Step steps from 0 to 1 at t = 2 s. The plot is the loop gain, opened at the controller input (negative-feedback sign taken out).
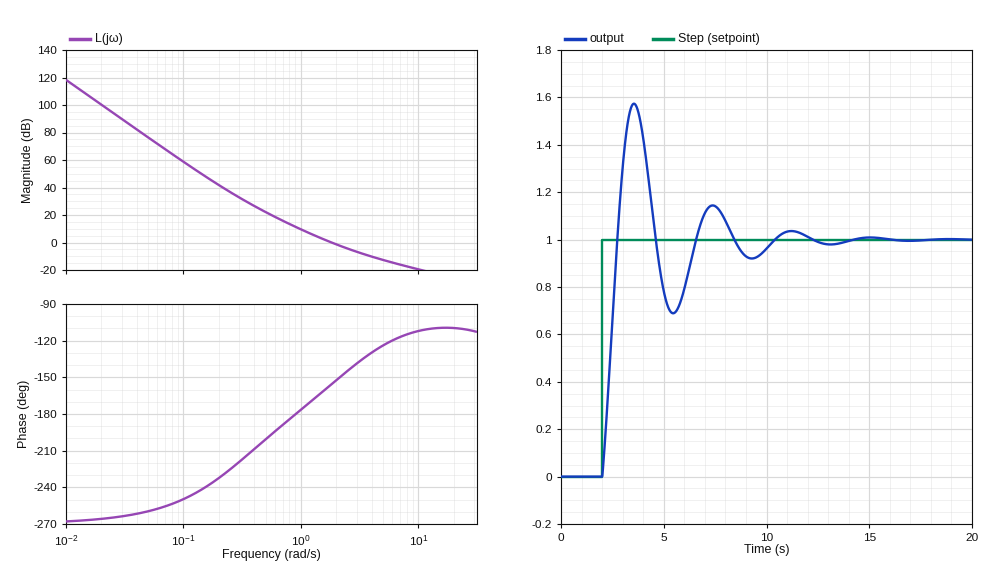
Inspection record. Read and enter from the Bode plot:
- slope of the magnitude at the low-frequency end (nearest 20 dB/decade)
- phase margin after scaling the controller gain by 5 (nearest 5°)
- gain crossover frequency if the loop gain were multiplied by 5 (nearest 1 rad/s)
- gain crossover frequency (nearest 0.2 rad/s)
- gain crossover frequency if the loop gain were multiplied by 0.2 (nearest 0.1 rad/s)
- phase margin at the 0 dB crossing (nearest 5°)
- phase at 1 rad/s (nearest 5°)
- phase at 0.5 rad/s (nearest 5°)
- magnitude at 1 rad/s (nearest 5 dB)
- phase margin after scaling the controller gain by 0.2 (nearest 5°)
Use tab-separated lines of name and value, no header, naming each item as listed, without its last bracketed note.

slope of the magnitude at the low-frequency end	-60 dB/decade
phase margin after scaling the controller gain by 5	60°
gain crossover frequency if the loop gain were multiplied by 5	6 rad/s
gain crossover frequency	1.8 rad/s
gain crossover frequency if the loop gain were multiplied by 0.2	0.8 rad/s
phase margin at the 0 dB crossing	25°
phase at 1 rad/s	-175°
phase at 0.5 rad/s	-200°
magnitude at 1 rad/s	10 dB
phase margin after scaling the controller gain by 0.2	-5°
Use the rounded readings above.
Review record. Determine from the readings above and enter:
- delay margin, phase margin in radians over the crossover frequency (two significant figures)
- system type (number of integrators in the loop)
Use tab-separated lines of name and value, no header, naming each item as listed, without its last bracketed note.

delay margin, phase margin in radians over the crossover frequency	0.24 s
system type	3
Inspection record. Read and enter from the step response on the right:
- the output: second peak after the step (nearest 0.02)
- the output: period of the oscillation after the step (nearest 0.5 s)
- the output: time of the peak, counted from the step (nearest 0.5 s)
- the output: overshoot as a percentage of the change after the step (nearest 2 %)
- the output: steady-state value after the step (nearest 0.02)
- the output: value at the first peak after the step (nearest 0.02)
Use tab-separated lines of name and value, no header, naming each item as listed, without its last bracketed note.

the output: second peak after the step	1.14
the output: period of the oscillation after the step	4.0 s
the output: time of the peak, counted from the step	1.5 s
the output: overshoot as a percentage of the change after the step	58 %
the output: steady-state value after the step	1.00
the output: value at the first peak after the step	1.58
